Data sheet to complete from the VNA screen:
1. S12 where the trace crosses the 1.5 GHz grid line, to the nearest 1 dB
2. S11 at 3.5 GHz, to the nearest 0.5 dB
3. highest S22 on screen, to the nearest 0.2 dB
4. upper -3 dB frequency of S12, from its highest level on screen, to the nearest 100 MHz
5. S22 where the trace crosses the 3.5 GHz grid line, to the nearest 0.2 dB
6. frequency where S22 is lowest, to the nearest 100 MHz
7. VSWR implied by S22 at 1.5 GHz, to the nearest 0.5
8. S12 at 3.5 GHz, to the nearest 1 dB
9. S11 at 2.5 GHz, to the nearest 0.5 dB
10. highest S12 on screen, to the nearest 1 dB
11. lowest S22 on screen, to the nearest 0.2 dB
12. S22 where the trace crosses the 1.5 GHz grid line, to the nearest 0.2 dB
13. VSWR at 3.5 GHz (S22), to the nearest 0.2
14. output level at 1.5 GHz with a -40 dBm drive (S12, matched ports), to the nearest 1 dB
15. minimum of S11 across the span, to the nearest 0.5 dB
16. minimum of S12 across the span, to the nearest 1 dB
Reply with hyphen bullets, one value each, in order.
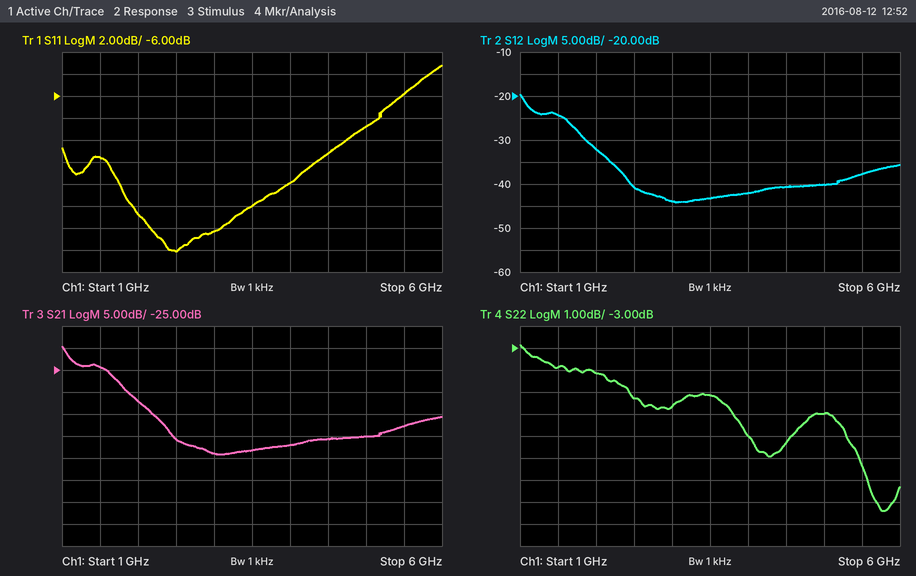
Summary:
- -24 dB
- -16.0 dB
- -2.8 dB
- 1.1 GHz
- -5.2 dB
- 5.8 GHz
- 4.5
- -43 dB
- -20.0 dB
- -20 dB
- -10.4 dB
- -3.8 dB
- 3.4
- -64 dBm
- -20.0 dB
- -44 dB
